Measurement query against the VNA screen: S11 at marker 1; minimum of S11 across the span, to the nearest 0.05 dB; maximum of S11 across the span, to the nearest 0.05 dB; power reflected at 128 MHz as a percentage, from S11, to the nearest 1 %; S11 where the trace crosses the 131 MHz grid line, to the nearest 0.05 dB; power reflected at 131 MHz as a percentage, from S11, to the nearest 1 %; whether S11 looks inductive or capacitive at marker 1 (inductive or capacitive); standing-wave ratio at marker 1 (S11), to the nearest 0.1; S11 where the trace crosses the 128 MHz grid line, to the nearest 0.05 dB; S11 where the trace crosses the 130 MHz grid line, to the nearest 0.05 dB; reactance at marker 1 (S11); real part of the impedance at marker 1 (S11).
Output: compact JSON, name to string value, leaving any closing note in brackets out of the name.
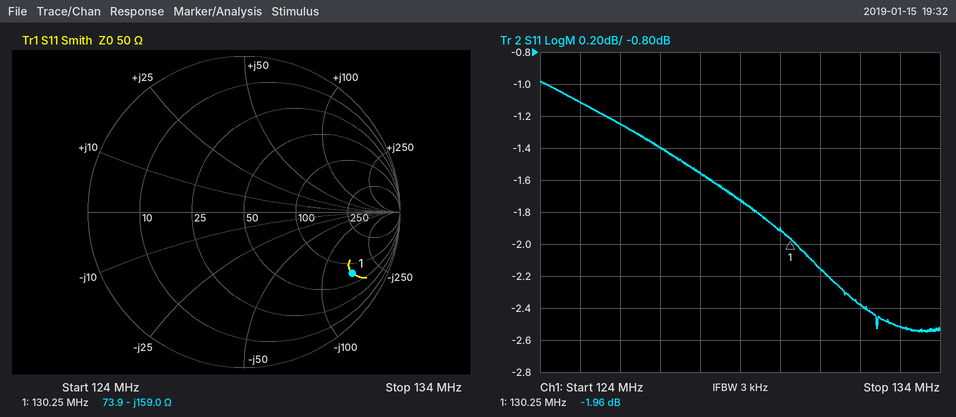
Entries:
{"S11 at marker 1": "-1.96 dB", "minimum of S11 across the span, to the nearest 0.05 dB": "-2.55 dB", "maximum of S11 across the span, to the nearest 0.05 dB": "-1.00 dB", "power reflected at 128 MHz as a percentage, from S11, to the nearest 1 %": "70 %", "S11 where the trace crosses the 131 MHz grid line, to the nearest 0.05 dB": "-2.15 dB", "power reflected at 131 MHz as a percentage, from S11, to the nearest 1 %": "61 %", "whether S11 looks inductive or capacitive at marker 1": "capacitive", "standing-wave ratio at marker 1 (S11), to the nearest 0.1": "8.9", "S11 where the trace crosses the 128 MHz grid line, to the nearest 0.05 dB": "-1.55 dB", "S11 where the trace crosses the 130 MHz grid line, to the nearest 0.05 dB": "-1.90 dB", "reactance at marker 1": "-159.0 Ω", "real part of the impedance at marker 1": "73.9 Ω"}
